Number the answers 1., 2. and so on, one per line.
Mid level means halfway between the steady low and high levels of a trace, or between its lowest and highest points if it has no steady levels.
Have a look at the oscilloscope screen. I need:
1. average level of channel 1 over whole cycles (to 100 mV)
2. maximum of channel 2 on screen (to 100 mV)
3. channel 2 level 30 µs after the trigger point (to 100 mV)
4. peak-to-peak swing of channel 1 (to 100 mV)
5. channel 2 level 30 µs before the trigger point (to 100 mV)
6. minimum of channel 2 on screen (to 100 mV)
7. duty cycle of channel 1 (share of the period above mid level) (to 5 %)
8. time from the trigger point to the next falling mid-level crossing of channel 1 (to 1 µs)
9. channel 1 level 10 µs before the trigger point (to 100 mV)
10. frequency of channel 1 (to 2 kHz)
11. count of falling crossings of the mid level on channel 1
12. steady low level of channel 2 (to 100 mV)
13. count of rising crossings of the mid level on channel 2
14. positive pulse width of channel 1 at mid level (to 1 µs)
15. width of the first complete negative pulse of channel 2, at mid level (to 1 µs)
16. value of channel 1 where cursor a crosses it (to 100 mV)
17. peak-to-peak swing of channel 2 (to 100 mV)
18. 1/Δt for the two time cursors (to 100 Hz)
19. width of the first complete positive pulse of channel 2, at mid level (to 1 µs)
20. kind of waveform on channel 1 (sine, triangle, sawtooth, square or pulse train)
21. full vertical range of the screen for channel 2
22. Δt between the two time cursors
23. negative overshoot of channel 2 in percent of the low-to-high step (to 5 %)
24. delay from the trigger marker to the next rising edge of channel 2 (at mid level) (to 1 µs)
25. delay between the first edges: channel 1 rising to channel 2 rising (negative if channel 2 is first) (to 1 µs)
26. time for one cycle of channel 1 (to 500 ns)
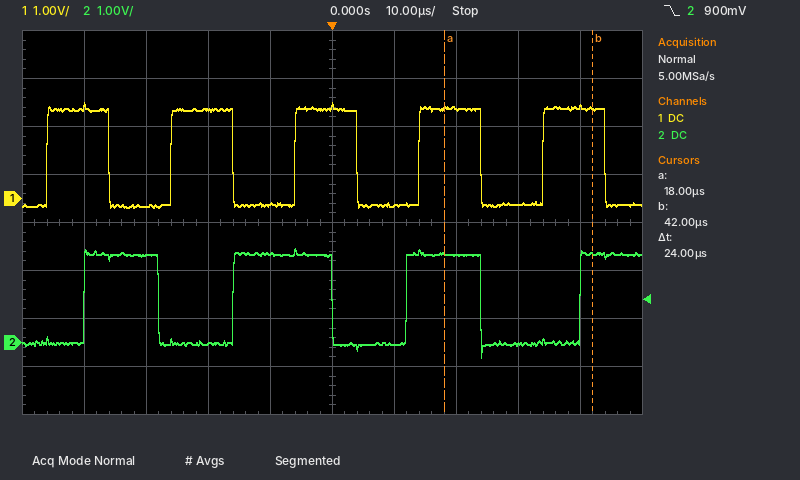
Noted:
1. 900 mV
2. 2.0 V
3. 0.0 V
4. 2.2 V
5. 1.8 V
6. -300 mV
7. 50 %
8. 4 µs
9. -100 mV
10. 50 kHz
11. 5
12. 0.0 V
13. 4
14. 10 µs
15. 12 µs
16. 1.9 V
17. 2.3 V
18. 41.7 kHz
19. 12 µs
20. square
21. 8 V
22. 24 µs
23. 15 %
24. 12 µs
25. +6 µs
26. 20.0 µs
